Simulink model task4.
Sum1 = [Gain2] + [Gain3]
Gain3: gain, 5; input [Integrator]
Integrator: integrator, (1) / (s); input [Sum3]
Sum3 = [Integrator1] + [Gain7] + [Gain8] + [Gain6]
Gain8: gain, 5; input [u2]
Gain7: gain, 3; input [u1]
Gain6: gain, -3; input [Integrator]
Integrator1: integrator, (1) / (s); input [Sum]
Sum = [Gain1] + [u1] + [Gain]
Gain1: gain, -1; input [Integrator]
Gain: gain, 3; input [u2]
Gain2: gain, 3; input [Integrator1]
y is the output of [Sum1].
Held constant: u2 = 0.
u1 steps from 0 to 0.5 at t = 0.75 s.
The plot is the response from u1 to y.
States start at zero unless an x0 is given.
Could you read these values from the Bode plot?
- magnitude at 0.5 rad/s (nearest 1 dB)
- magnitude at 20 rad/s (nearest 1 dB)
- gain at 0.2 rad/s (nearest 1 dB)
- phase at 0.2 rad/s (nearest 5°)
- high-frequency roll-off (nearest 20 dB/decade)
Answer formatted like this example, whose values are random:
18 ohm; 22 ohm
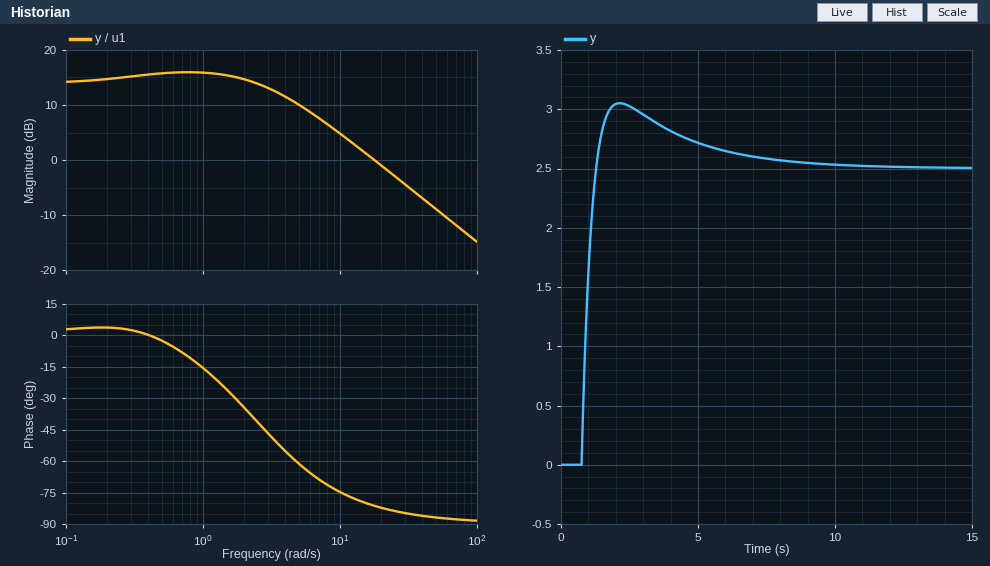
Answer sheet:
16 dB; -1 dB; 15 dB; 5°; -20 dB/decade
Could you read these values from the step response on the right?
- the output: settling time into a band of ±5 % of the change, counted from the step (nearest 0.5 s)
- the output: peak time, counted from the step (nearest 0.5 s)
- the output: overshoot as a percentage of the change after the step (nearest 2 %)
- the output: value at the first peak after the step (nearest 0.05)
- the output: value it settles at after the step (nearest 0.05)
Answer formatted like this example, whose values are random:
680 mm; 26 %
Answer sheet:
5.5 s; 1.5 s; 22 %; 3.05; 2.50
